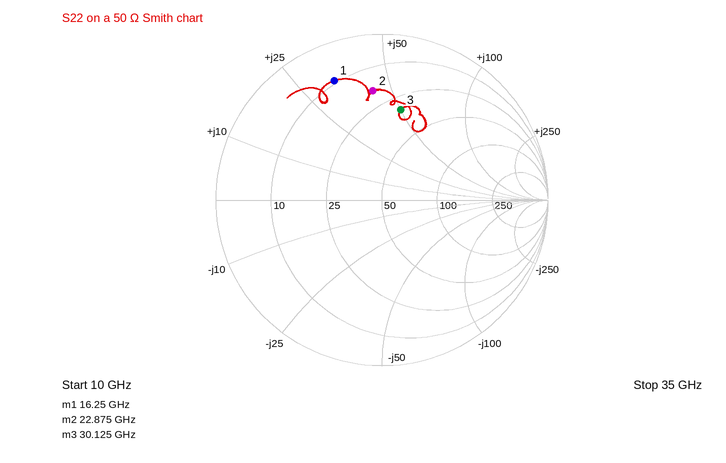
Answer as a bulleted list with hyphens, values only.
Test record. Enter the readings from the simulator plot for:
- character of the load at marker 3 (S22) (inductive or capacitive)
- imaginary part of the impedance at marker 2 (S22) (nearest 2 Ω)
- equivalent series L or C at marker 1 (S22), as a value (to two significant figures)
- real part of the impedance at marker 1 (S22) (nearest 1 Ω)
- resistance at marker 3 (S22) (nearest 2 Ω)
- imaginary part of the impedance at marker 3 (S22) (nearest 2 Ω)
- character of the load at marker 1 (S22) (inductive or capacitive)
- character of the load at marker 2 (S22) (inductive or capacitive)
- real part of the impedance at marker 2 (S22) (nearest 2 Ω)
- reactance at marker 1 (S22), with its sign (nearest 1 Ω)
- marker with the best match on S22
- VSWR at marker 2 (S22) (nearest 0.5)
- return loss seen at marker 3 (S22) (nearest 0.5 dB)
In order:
- inductive
- +42 Ω
- 320 pH
- 9 Ω
- 32 Ω
- +50 Ω
- inductive
- inductive
- 18 Ω
- +33 Ω
- marker 3
- 5.0
- 5.0 dB
